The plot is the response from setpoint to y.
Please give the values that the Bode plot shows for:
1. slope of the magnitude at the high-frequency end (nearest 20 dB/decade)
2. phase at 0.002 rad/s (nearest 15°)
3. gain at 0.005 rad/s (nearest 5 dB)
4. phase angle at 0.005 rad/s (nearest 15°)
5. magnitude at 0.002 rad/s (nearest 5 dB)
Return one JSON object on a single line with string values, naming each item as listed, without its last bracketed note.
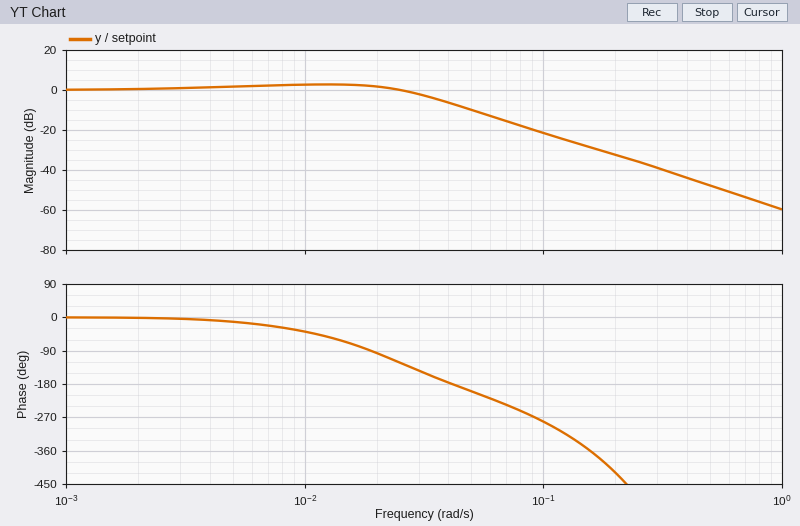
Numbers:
{"slope of the magnitude at the high-frequency end": "-40 dB/decade", "phase at 0.002 rad/s": "0°", "gain at 0.005 rad/s": "0 dB", "phase angle at 0.005 rad/s": "-15°", "magnitude at 0.002 rad/s": "0 dB"}
